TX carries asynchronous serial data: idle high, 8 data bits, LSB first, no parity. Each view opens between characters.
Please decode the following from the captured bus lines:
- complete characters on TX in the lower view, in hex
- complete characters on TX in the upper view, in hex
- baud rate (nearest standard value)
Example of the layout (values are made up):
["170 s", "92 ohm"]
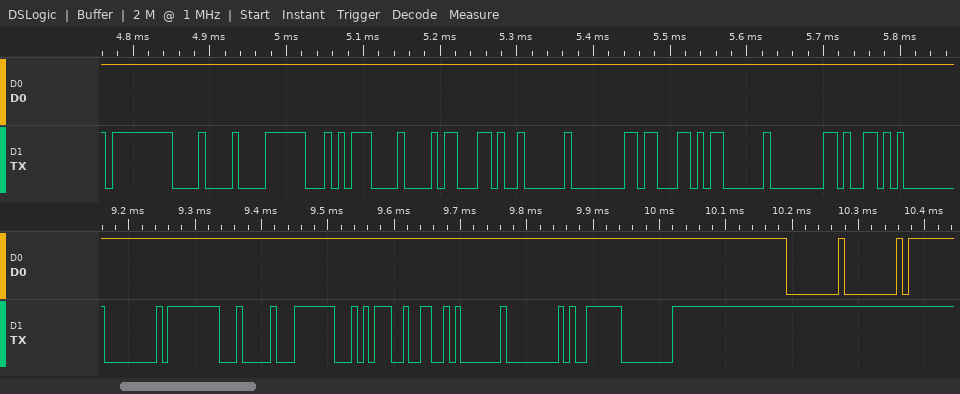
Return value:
["00, FF, 04, FC, D4, 32, 01, 00, F9, 00", "FF, 08, F8, D4, 08, 63, 02, 80, 63, 03, 80, 59", "115200 baud"]
